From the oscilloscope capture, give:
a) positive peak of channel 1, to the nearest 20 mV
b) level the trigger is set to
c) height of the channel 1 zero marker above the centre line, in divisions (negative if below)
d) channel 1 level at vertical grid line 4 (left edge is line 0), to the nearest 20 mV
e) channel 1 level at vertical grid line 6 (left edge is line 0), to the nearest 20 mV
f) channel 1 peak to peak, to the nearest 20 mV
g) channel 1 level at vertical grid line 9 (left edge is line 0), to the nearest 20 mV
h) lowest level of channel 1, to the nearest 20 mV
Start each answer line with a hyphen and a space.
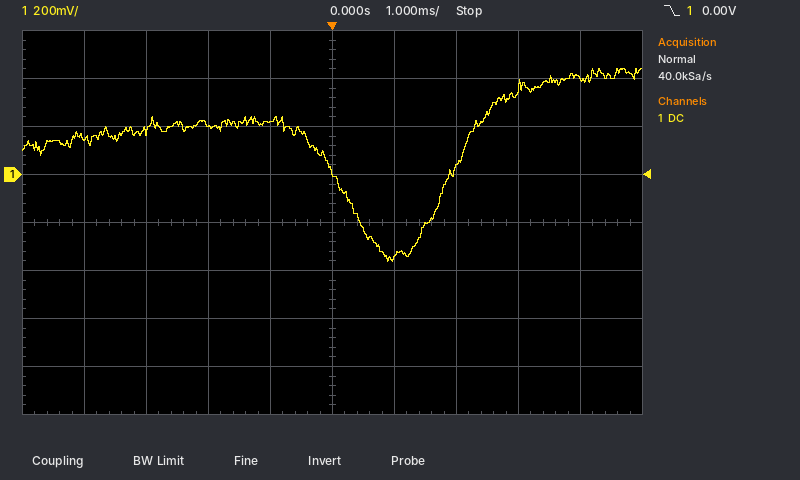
- 440 mV
- 0.00 V
- +1.0 div
- 220 mV
- -340 mV
- 800 mV
- 400 mV
- -360 mV
